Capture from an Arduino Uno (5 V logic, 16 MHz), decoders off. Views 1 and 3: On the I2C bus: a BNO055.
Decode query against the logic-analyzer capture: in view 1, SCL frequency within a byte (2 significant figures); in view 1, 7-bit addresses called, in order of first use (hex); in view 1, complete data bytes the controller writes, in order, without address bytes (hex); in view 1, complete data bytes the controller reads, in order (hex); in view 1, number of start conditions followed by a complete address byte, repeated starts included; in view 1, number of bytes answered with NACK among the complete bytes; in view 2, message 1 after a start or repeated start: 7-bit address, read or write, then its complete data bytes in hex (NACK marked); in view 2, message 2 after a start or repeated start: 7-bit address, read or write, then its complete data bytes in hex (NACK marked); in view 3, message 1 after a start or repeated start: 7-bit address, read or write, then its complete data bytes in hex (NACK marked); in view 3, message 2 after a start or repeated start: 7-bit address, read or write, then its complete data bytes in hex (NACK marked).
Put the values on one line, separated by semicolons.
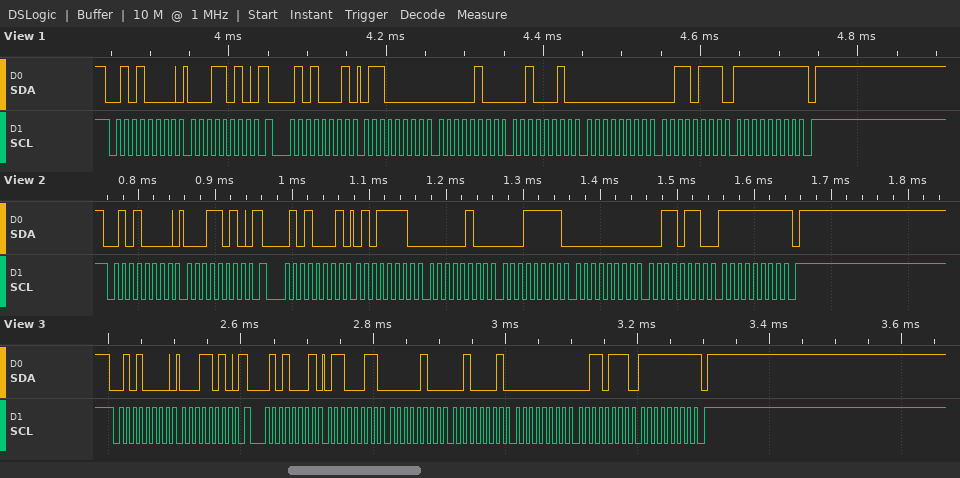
100 kHz; 0x28; 1A; 60 04 22 00 37 FF; 2; 1; 0x28 write: 1A; 0x28 read: 5E 04 1F 00 36 FF NACK; 0x28 write: 1A; 0x28 read: 63 04 21 00 37 FF NACK
